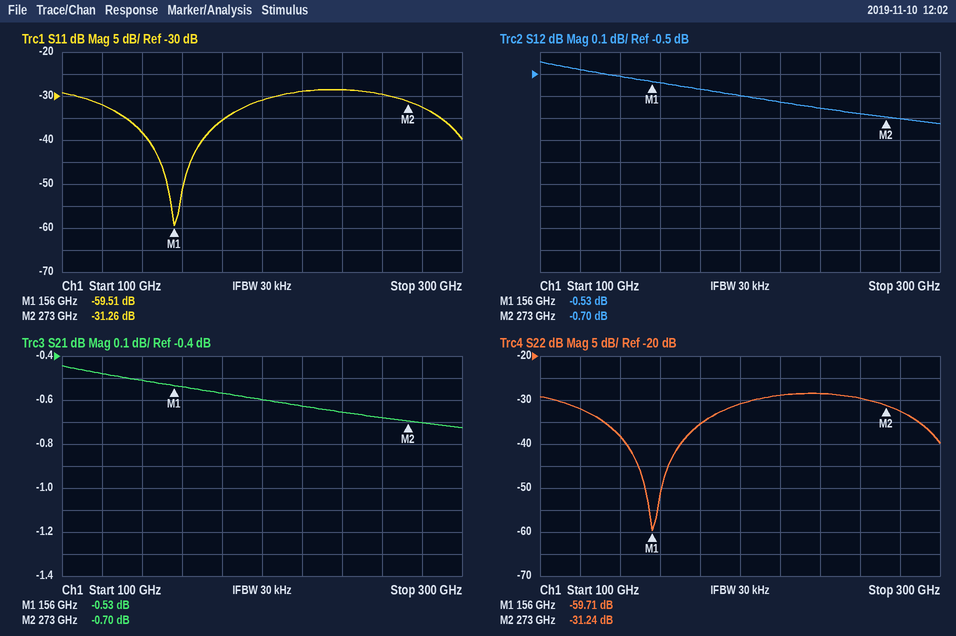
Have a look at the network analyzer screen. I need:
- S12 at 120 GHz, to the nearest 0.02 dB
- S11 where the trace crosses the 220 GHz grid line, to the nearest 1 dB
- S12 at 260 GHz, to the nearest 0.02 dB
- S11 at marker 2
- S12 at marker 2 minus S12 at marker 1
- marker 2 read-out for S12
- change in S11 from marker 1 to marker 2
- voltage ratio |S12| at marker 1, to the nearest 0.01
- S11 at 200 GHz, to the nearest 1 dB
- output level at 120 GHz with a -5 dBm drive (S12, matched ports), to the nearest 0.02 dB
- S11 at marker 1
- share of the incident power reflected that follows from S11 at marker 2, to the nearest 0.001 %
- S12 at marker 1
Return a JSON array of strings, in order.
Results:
["-0.48 dB", "-29 dB", "-0.68 dB", "-31.26 dB", "-0.17 dB", "-0.70 dB", "28.25 dB", "0.94", "-31 dB", "-5.48 dBm", "-59.51 dB", "0.075 %", "-0.53 dB"]
